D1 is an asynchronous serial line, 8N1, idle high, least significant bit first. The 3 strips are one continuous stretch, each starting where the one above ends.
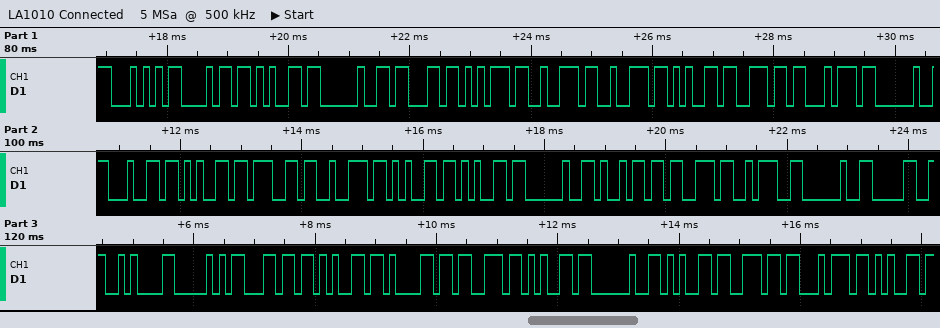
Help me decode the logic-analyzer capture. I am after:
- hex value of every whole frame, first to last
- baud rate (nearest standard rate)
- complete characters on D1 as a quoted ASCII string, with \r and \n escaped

54 68 65 20 63 75 72 72 65 6E 74 20 64 65 67 72 65 65 20 69 73 3A 20 30 0A 50 6C 65 61 73 65 20 65 6E 74 65
9600 baud
"The current degree is: 0\nPlease ente"
